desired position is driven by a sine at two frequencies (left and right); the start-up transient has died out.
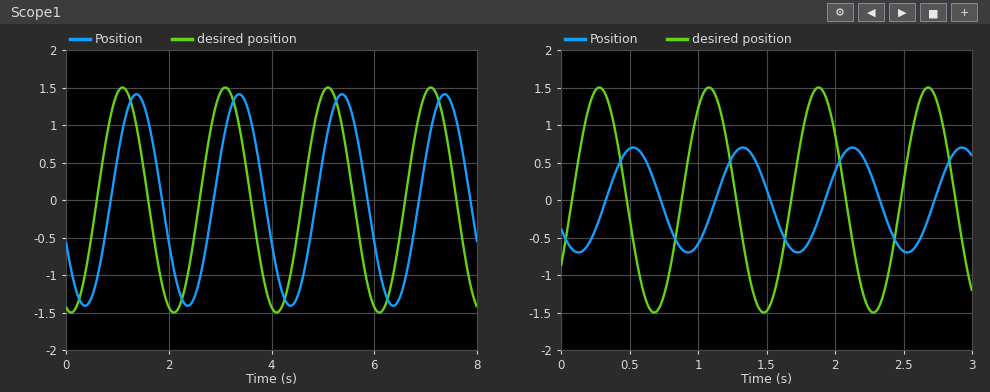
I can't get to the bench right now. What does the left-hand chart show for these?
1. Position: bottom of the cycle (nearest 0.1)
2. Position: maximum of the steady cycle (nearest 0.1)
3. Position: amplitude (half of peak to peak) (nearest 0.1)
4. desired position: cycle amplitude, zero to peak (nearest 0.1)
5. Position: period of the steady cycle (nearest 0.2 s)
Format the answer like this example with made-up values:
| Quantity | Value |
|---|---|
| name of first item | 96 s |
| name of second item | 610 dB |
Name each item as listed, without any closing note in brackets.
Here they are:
| Quantity | Value |
|---|---|
| Position: bottom of the cycle | -1.4 |
| Position: maximum of the steady cycle | 1.4 |
| Position: amplitude (half of peak to peak) | 1.4 |
| desired position: cycle amplitude, zero to peak | 1.5 |
| Position: period of the steady cycle | 2.0 s |
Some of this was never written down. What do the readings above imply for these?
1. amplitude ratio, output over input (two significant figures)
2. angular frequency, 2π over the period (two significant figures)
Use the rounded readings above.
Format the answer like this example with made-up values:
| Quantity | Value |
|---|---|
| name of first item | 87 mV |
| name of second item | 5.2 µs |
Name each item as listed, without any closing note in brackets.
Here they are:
| Quantity | Value |
|---|---|
| amplitude ratio, output over input | 0.93 |
| angular frequency, 2π over the period | 3.1 rad/s |
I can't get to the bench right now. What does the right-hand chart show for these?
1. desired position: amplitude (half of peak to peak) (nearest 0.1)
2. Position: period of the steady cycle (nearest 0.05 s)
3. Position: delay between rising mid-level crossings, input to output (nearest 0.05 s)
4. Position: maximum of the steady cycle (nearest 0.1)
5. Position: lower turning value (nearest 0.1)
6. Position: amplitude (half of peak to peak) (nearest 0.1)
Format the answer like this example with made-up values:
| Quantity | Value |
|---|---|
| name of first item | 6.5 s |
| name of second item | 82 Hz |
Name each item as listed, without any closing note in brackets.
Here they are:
| Quantity | Value |
|---|---|
| desired position: amplitude (half of peak to peak) | 1.5 |
| Position: period of the steady cycle | 0.80 s |
| Position: delay between rising mid-level crossings, input to output | 0.25 s |
| Position: maximum of the steady cycle | 0.7 |
| Position: lower turning value | -0.7 |
| Position: amplitude (half of peak to peak) | 0.7 |
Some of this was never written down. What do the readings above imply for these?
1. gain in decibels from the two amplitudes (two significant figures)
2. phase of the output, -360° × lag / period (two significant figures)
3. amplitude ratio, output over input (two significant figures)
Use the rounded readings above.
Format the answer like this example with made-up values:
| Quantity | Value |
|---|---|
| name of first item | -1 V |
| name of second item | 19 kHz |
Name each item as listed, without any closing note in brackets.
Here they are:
| Quantity | Value |
|---|---|
| gain in decibels from the two amplitudes | -6.6 dB |
| phase of the output, -360° × lag / period | -110° |
| amplitude ratio, output over input | 0.47 |
